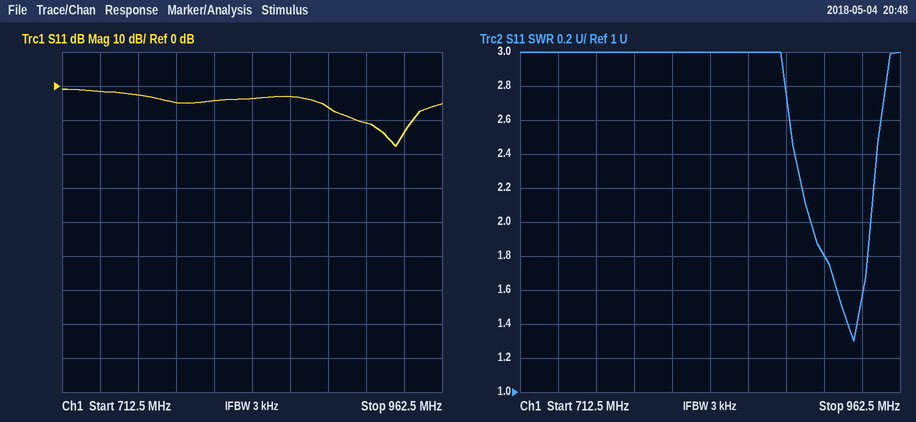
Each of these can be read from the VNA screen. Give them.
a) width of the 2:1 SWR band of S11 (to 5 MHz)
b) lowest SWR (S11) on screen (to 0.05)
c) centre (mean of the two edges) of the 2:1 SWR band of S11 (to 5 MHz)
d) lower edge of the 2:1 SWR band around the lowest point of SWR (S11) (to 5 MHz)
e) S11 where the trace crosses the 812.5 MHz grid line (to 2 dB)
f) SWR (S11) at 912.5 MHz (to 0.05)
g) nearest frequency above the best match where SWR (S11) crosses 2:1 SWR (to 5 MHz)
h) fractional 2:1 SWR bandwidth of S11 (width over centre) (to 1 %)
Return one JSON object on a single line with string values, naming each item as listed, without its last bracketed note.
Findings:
{"width of the 2:1 SWR band of S11": "40 MHz", "lowest SWR (S11) on screen": "1.30", "centre (mean of the two edges) of the 2:1 SWR band of S11": "925 MHz", "lower edge of the 2:1 SWR band around the lowest point of SWR (S11)": "905 MHz", "S11 where the trace crosses the 812.5 MHz grid line": "-4 dB", "SWR (S11) at 912.5 MHz": "1.80", "nearest frequency above the best match where SWR (S11) crosses 2:1 SWR": "945 MHz", "fractional 2:1 SWR bandwidth of S11 (width over centre)": "4 %"}
